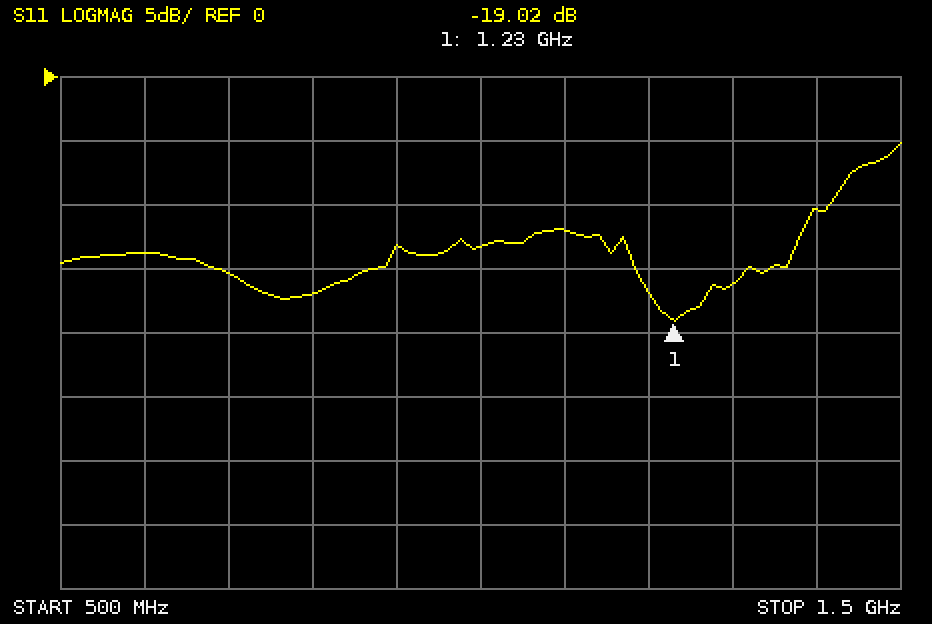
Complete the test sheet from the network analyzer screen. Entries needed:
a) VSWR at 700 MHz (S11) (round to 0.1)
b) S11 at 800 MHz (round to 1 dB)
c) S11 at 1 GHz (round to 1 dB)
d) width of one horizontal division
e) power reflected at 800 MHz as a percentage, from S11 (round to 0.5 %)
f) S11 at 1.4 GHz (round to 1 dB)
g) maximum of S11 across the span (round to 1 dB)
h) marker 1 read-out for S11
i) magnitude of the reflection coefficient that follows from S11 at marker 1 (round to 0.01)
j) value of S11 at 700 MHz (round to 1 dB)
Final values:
1.4
-17 dB
-13 dB
100 MHz
2.0 %
-10 dB
-5 dB
-19.02 dB
0.11
-15 dB
